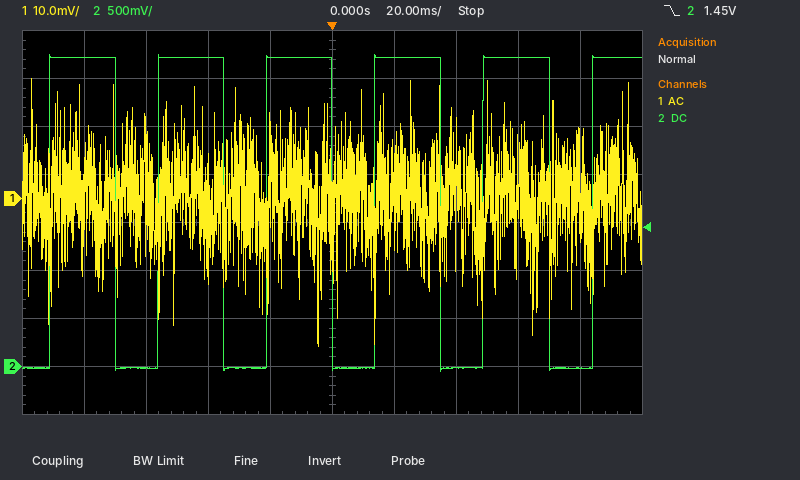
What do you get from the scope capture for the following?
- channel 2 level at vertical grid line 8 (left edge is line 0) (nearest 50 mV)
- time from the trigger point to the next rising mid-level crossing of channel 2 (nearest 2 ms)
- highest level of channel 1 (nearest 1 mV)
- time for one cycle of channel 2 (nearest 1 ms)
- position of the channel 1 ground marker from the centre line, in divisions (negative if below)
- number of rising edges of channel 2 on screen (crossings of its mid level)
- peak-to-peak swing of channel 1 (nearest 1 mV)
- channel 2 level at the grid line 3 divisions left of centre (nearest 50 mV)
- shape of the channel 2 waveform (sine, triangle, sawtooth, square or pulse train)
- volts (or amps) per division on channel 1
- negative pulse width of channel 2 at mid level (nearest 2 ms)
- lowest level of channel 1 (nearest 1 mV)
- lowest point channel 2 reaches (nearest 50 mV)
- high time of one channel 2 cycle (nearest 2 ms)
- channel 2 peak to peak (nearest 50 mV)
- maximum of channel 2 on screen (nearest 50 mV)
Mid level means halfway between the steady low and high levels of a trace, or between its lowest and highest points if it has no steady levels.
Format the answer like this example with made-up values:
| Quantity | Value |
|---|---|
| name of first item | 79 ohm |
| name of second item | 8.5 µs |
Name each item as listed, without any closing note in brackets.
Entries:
| Quantity | Value |
|---|---|
| channel 2 level at vertical grid line 8 (left edge is line 0) | 3.20 V |
| time from the trigger point to the next rising mid-level crossing of channel 2 | 14 ms |
| highest level of channel 1 | 25 mV |
| time for one cycle of channel 2 | 35 ms |
| position of the channel 1 ground marker from the centre line, in divisions | +0.5 div |
| number of rising edges of channel 2 on screen | 6 |
| peak-to-peak swing of channel 1 | 56 mV |
| channel 2 level at the grid line 3 divisions left of centre | 0 mV |
| shape of the channel 2 waveform | pulse train |
| volts (or amps) per division on channel 1 | 10 mV |
| negative pulse width of channel 2 at mid level | 14 ms |
| lowest level of channel 1 | -31 mV |
| lowest point channel 2 reaches | -50 mV |
| high time of one channel 2 cycle | 22 ms |
| channel 2 peak to peak | 3.30 V |
| maximum of channel 2 on screen | 3.25 V |
